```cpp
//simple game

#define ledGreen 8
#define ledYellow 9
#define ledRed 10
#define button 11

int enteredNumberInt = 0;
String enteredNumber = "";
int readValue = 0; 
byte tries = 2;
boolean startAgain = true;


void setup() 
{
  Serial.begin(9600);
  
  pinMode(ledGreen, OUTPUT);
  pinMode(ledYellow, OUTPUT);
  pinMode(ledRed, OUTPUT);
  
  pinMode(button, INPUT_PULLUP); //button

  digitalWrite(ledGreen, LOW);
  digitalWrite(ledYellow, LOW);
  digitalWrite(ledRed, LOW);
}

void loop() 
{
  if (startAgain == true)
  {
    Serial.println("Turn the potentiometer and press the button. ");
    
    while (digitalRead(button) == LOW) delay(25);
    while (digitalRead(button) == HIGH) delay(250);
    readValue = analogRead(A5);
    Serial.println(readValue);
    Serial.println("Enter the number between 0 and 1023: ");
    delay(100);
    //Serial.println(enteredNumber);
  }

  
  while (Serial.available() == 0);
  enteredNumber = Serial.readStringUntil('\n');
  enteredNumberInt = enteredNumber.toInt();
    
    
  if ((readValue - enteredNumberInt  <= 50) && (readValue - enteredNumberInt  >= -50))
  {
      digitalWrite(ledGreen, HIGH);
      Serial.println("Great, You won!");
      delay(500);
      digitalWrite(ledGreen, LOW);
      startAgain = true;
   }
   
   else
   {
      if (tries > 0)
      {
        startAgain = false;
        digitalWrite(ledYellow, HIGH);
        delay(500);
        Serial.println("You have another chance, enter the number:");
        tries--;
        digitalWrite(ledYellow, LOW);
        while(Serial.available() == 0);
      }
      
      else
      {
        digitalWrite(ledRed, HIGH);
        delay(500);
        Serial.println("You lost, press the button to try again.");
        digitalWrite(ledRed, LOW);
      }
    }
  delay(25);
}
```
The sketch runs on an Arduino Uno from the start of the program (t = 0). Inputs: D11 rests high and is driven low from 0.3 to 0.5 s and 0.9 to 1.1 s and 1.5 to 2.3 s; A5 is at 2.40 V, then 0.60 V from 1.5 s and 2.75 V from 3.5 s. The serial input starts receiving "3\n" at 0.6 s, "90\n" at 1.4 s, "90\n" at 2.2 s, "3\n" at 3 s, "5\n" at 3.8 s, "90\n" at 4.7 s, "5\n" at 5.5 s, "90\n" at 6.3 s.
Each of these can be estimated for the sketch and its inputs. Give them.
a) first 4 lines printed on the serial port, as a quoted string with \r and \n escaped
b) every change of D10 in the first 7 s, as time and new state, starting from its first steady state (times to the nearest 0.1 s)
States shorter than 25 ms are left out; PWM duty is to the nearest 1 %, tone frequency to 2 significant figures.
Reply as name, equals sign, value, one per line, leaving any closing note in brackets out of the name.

first 4 lines printed on the serial port, as a quoted string with \r and \n escaped = "Turn the potentiometer and press the button. \r\n491\r\nEnter the number between 0 and 1023: \r\nYou have another chance, enter the number:\r\n"
every change of D10 in the first 7 s, as time and new state, starting from its first steady state = 0 s low; 2.2 s high; 2.7 s low; 3 s high; 3.5 s low; 3.8 s high; 4.3 s low; 4.7 s high; 5.2 s low; 5.5 s high; 6 s low; 6.3 s high; 6.8 s low
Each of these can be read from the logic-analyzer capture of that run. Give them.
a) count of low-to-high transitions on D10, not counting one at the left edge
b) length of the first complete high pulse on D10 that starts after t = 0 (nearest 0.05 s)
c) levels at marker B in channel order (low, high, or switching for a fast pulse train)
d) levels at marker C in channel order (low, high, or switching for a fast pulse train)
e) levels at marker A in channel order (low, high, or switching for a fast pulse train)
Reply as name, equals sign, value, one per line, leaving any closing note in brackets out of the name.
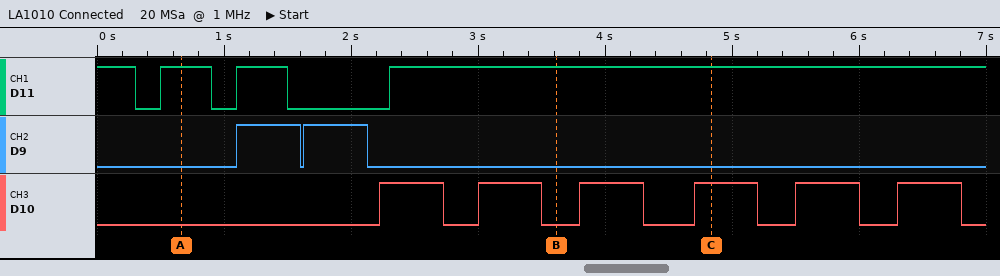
count of low-to-high transitions on D10, not counting one at the left edge = 6
length of the first complete high pulse on D10 that starts after t = 0 = 0.50 s
levels at marker B in channel order = D11 high, D9 low, D10 low
levels at marker C in channel order = D11 high, D9 low, D10 high
levels at marker A in channel order = D11 high, D9 low, D10 low
